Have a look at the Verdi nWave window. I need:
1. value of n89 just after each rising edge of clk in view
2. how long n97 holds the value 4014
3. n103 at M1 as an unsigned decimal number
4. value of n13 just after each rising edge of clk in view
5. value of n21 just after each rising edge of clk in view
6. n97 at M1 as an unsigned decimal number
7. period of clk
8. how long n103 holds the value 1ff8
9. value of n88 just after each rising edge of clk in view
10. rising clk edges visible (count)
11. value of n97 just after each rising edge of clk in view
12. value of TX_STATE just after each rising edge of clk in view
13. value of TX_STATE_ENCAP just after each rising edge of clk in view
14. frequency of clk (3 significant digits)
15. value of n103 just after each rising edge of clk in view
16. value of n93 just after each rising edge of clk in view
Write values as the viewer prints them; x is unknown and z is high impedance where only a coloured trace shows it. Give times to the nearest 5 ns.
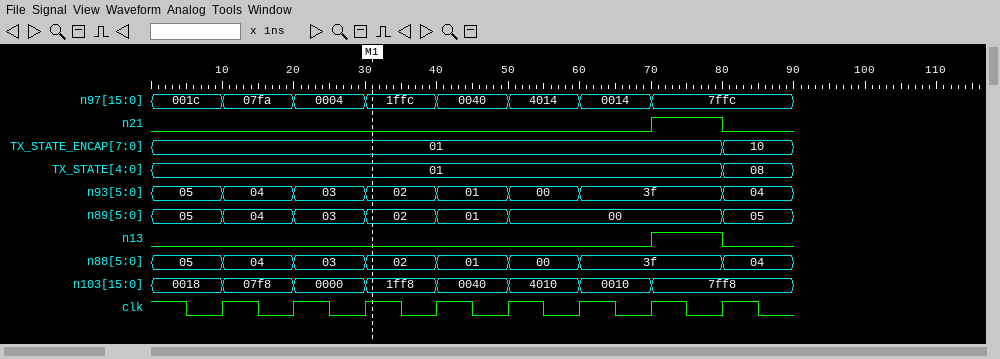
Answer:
04, 03, 02, 01, 00, 00, 00, 05
10 ns
8184
0 0 0 0 0 0 1 0
0 0 0 0 0 0 1 0
8188
10 ns
10 ns
04, 03, 02, 01, 00, 3f, 3f, 04
8
07fa, 0004, 1ffc, 0040, 4014, 0014, 7ffc, 7ffc
01, 01, 01, 01, 01, 01, 01, 08
01, 01, 01, 01, 01, 01, 01, 10
100 MHz
07f8, 0000, 1ff8, 0040, 4010, 0010, 7ff8, 7ff8
04, 03, 02, 01, 00, 3f, 3f, 04
